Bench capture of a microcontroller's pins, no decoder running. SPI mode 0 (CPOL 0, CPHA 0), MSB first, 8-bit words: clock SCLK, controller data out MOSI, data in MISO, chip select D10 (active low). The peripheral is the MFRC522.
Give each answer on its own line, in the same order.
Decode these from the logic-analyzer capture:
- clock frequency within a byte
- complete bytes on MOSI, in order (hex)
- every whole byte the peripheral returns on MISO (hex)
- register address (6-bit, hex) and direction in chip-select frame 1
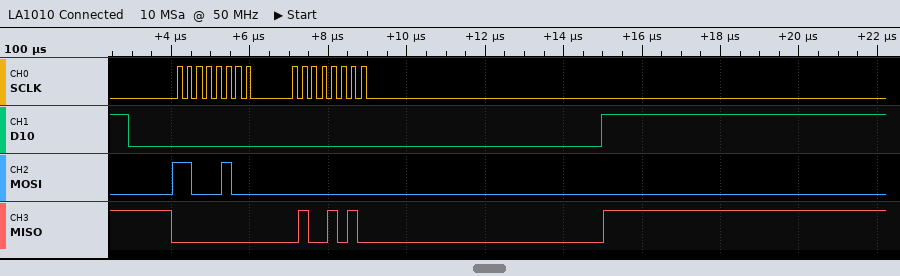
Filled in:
4 MHz
0xC4 0x00
0x00 0x4A
0x22 read
